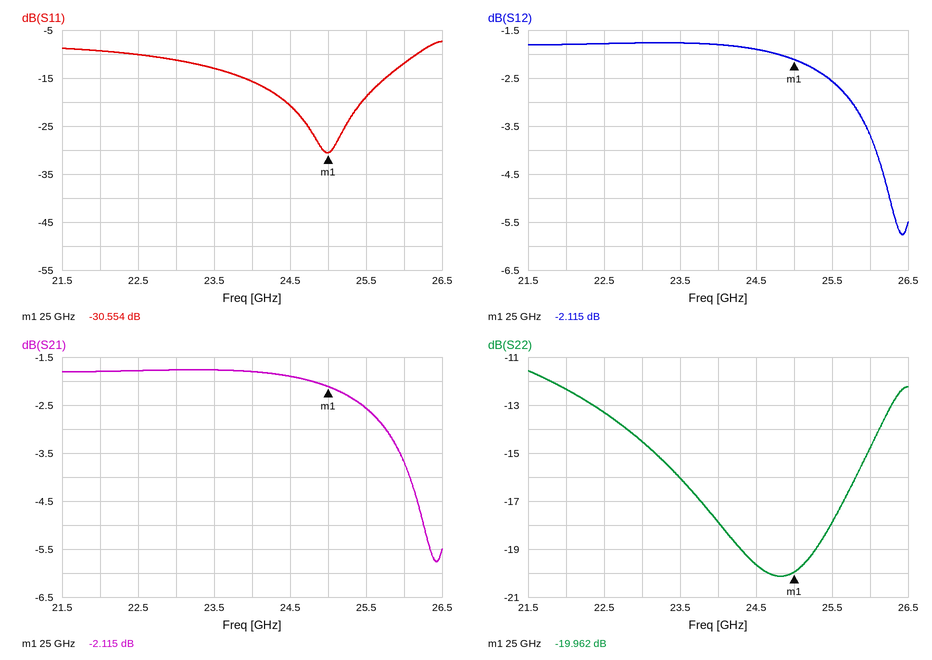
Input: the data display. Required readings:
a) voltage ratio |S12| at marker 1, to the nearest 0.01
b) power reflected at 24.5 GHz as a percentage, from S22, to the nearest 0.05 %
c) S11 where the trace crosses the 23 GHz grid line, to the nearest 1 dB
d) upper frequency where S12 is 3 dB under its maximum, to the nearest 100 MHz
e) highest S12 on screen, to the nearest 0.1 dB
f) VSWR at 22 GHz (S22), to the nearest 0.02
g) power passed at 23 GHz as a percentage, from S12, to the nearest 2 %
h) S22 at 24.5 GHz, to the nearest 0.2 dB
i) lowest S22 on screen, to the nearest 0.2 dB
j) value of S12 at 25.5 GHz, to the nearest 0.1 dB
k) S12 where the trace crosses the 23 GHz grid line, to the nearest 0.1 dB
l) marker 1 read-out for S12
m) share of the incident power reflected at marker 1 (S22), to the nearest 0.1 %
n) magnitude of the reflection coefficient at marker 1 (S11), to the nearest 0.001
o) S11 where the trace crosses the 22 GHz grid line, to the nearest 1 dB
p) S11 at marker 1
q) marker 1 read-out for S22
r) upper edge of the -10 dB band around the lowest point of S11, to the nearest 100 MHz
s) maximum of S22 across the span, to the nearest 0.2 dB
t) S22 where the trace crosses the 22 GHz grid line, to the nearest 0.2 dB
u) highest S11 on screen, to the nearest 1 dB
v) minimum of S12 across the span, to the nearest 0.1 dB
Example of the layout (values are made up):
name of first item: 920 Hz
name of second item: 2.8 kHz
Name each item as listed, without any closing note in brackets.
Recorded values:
voltage ratio |S12| at marker 1, to the nearest 0.01: 0.78
power reflected at 24.5 GHz as a percentage, from S22, to the nearest 0.05 %: 1.10 %
S11 where the trace crosses the 23 GHz grid line, to the nearest 1 dB: -11 dB
upper frequency where S12 is 3 dB under its maximum, to the nearest 100 MHz: 26.2 GHz
highest S12 on screen, to the nearest 0.1 dB: -1.8 dB
VSWR at 22 GHz (S22), to the nearest 0.02: 1.64
power passed at 23 GHz as a percentage, from S12, to the nearest 2 %: 66 %
S22 at 24.5 GHz, to the nearest 0.2 dB: -19.6 dB
lowest S22 on screen, to the nearest 0.2 dB: -20.2 dB
value of S12 at 25.5 GHz, to the nearest 0.1 dB: -2.6 dB
S12 where the trace crosses the 23 GHz grid line, to the nearest 0.1 dB: -1.8 dB
marker 1 read-out for S12: -2.115 dB
share of the incident power reflected at marker 1 (S22), to the nearest 0.1 %: 1.0 %
magnitude of the reflection coefficient at marker 1 (S11), to the nearest 0.001: 0.030
S11 where the trace crosses the 22 GHz grid line, to the nearest 1 dB: -9 dB
S11 at marker 1: -30.554 dB
marker 1 read-out for S22: -19.962 dB
upper edge of the -10 dB band around the lowest point of S11, to the nearest 100 MHz: 26.2 GHz
maximum of S22 across the span, to the nearest 0.2 dB: -11.6 dB
S22 where the trace crosses the 22 GHz grid line, to the nearest 0.2 dB: -12.4 dB
highest S11 on screen, to the nearest 1 dB: -7 dB
minimum of S12 across the span, to the nearest 0.1 dB: -5.8 dB
